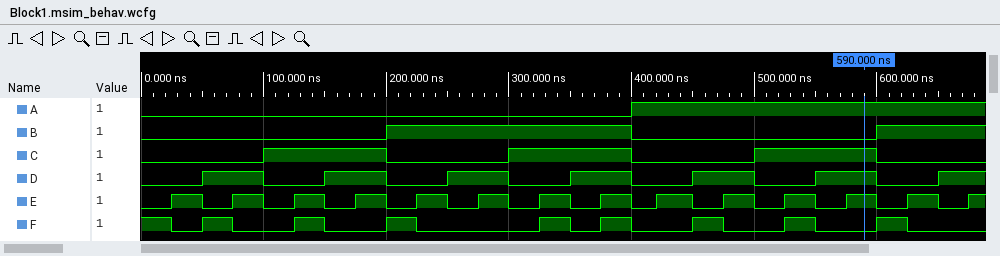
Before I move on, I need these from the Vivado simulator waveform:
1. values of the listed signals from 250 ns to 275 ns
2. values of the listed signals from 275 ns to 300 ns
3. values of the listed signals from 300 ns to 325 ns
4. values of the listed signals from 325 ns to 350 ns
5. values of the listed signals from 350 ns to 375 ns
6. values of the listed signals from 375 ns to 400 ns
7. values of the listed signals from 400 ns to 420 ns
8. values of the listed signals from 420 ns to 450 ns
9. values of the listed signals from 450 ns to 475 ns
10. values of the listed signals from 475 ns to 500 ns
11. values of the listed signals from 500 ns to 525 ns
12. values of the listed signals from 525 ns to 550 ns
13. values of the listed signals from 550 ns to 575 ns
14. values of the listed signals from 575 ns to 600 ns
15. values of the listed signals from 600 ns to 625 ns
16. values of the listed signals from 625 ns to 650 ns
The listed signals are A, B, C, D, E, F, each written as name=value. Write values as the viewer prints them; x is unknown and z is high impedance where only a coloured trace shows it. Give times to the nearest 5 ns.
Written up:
A=0, B=1, C=0, D=1, E=0, F=0
A=0, B=1, C=0, D=1, E=1, F=0
A=0, B=1, C=1, D=0, E=0, F=0
A=0, B=1, C=1, D=0, E=1, F=1
A=0, B=1, C=1, D=1, E=0, F=0
A=0, B=1, C=1, D=1, E=1, F=1
A=1, B=0, C=0, D=0, E=0, F=0
A=1, B=0, C=0, D=0, E=1, F=0
A=1, B=0, C=0, D=1, E=0, F=1
A=1, B=0, C=0, D=1, E=1, F=0
A=1, B=0, C=1, D=0, E=0, F=0
A=1, B=0, C=1, D=0, E=1, F=1
A=1, B=0, C=1, D=1, E=0, F=0
A=1, B=0, C=1, D=1, E=1, F=0
A=1, B=1, C=0, D=0, E=0, F=1
A=1, B=1, C=0, D=0, E=1, F=0
